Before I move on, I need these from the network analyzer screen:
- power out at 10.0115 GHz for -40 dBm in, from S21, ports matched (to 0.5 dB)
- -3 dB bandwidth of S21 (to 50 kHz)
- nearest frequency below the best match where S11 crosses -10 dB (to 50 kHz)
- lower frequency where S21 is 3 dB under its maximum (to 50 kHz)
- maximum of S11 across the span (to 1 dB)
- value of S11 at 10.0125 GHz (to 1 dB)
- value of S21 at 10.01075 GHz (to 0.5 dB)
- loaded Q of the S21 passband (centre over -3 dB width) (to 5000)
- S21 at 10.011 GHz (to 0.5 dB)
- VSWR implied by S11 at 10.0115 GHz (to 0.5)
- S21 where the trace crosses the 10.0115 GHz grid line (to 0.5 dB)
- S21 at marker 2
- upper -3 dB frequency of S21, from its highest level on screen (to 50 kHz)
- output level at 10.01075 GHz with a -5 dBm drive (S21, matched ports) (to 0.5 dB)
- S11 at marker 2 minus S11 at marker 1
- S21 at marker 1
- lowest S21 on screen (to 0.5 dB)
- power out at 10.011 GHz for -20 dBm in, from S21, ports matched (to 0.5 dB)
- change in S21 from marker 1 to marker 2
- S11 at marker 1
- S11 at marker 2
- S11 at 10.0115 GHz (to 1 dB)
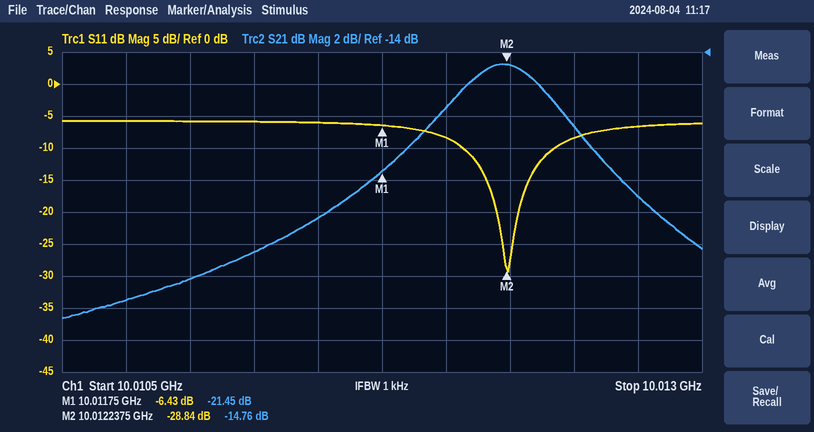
-64.5 dBm
450 kHz
10.01205 GHz
10.01200 GHz
-6 dB
-8 dB
-29.5 dB
20000
-28.0 dB
3.0
-24.5 dB
-14.76 dB
10.01245 GHz
-34.5 dBm
-22.41 dB
-21.45 dB
-30.5 dB
-48.0 dBm
6.69 dB
-6.43 dB
-28.84 dB
-6 dB
